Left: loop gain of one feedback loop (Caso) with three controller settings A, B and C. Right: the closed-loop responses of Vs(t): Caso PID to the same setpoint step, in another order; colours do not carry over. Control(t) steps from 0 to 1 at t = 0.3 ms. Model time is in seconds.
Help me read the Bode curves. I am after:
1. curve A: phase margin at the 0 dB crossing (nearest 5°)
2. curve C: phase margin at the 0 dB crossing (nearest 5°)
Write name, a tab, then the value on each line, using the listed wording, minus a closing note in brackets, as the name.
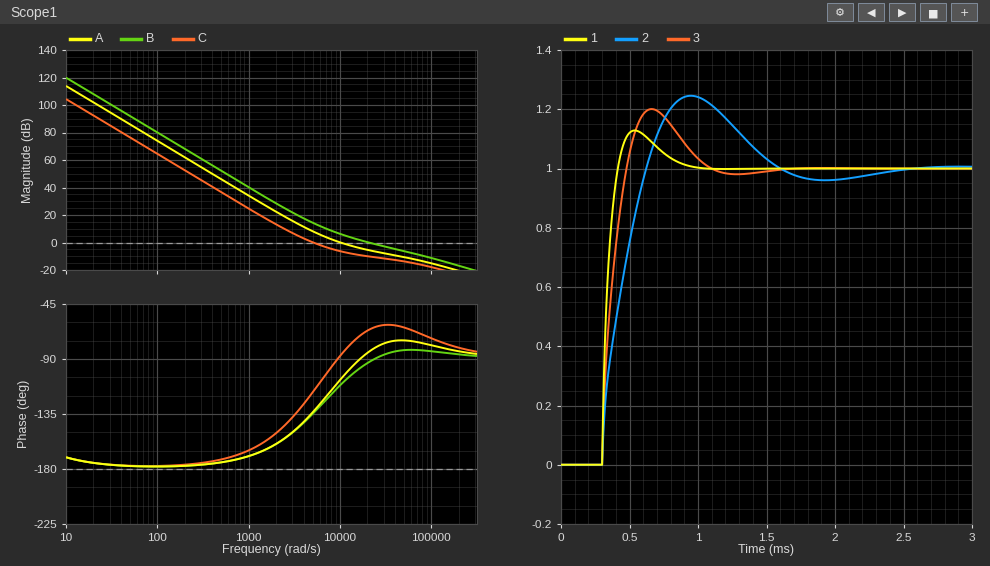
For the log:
curve A: phase margin at the 0 dB crossing	75°
curve C: phase margin at the 0 dB crossing	65°
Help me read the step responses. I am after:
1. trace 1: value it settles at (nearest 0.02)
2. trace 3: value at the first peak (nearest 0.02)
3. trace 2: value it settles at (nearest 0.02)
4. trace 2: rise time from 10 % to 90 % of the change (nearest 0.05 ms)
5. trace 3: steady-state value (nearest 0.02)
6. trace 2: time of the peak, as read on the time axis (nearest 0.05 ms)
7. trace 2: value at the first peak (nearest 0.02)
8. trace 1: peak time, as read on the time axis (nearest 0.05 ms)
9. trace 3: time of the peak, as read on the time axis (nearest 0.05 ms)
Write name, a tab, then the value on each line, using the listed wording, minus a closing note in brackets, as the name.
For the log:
trace 1: value it settles at	1.00
trace 3: value at the first peak	1.20
trace 2: value it settles at	1.00
trace 2: rise time from 10 % to 90 % of the change	0.25 ms
trace 3: steady-state value	1.00
trace 2: time of the peak, as read on the time axis	0.95 ms
trace 2: value at the first peak	1.24
trace 1: peak time, as read on the time axis	0.55 ms
trace 3: time of the peak, as read on the time axis	0.65 ms
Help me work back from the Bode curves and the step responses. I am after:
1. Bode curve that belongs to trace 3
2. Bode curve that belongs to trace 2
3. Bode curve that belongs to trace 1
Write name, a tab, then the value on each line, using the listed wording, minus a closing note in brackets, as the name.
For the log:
Bode curve that belongs to trace 3	A
Bode curve that belongs to trace 2	C
Bode curve that belongs to trace 1	B
